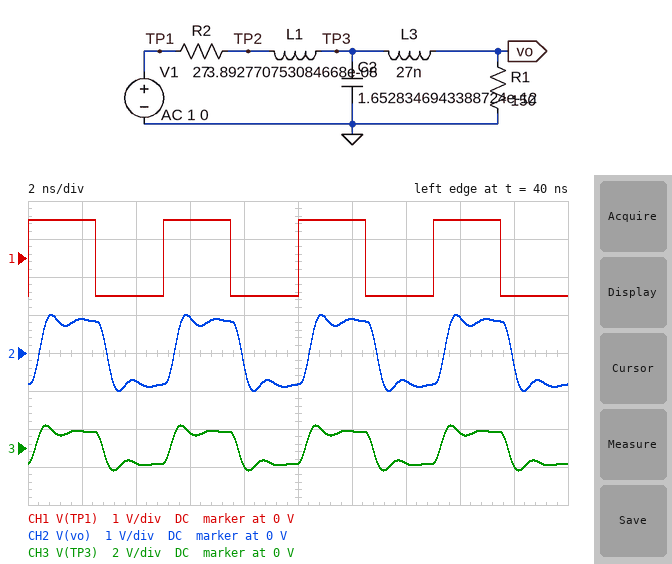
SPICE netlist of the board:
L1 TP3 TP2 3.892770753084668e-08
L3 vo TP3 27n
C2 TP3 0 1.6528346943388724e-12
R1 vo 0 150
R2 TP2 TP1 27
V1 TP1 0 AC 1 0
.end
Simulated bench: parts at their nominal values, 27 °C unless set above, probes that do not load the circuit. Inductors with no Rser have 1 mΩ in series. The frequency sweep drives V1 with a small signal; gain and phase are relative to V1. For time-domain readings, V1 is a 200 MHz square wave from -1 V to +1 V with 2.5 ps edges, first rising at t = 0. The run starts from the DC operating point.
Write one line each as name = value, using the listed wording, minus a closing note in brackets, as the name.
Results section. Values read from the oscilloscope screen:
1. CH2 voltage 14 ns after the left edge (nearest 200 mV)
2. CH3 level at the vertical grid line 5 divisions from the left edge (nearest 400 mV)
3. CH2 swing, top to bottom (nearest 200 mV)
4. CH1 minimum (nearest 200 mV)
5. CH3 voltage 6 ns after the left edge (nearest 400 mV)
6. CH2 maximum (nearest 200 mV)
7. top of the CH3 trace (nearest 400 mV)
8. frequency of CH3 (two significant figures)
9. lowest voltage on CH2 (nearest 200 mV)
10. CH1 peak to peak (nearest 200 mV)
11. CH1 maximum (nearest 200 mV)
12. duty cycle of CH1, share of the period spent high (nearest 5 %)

CH2 voltage 14 ns after the left edge = -800 mV
CH3 level at the vertical grid line 5 divisions from the left edge = -800 mV
CH2 swing, top to bottom = 2.0 V
CH1 minimum = -1.0 V
CH3 voltage 6 ns after the left edge = 800 mV
CH2 maximum = 1.0 V
top of the CH3 trace = 1.2 V
frequency of CH3 = 200 MHz
lowest voltage on CH2 = -1.0 V
CH1 peak to peak = 2.0 V
CH1 maximum = 1.0 V
duty cycle of CH1, share of the period spent high = 50 %
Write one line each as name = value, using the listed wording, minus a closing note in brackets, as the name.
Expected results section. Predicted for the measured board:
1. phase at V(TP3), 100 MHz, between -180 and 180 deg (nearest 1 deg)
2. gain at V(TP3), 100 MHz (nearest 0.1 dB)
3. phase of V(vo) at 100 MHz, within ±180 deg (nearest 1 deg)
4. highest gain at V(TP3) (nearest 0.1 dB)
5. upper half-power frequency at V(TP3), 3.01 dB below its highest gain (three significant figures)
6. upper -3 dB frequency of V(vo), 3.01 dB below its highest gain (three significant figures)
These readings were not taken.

phase at V(TP3), 100 MHz, between -180 and 180 deg = -8 deg
gain at V(TP3), 100 MHz = -1.5 dB
phase of V(vo) at 100 MHz, within ±180 deg = -15 deg
highest gain at V(TP3) = 1.3 dB
upper half-power frequency at V(TP3), 3.01 dB below its highest gain = 1.03 GHz
upper -3 dB frequency of V(vo), 3.01 dB below its highest gain = 988 MHz
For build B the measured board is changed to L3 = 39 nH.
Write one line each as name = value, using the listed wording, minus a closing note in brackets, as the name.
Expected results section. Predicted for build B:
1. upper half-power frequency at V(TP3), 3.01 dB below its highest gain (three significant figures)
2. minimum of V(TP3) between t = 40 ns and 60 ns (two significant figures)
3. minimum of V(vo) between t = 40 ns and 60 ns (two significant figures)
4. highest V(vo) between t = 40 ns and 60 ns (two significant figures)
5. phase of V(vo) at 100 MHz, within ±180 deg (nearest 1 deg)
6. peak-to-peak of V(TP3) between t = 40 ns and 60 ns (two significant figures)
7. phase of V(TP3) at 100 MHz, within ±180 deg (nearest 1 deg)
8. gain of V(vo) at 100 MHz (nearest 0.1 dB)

upper half-power frequency at V(TP3), 3.01 dB below its highest gain = 965 MHz
minimum of V(TP3) between t = 40 ns and 60 ns = -1.3 V
minimum of V(vo) between t = 40 ns and 60 ns = -960 mV
highest V(vo) between t = 40 ns and 60 ns = 960 mV
phase of V(vo) at 100 MHz, within ±180 deg = -17 deg
peak-to-peak of V(TP3) between t = 40 ns and 60 ns = 2.6 V
phase of V(TP3) at 100 MHz, within ±180 deg = -8 deg
gain of V(vo) at 100 MHz = -1.6 dB
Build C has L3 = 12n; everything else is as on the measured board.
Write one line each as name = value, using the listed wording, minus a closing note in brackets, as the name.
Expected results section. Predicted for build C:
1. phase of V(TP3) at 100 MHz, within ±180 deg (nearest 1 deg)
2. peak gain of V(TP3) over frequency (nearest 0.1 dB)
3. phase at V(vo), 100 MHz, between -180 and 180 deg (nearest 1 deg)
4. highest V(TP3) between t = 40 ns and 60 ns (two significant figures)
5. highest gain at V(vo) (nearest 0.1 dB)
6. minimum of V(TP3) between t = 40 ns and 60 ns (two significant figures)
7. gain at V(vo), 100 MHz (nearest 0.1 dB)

phase of V(TP3) at 100 MHz, within ±180 deg = -9 deg
peak gain of V(TP3) over frequency = -1.1 dB
phase at V(vo), 100 MHz, between -180 and 180 deg = -12 deg
highest V(TP3) between t = 40 ns and 60 ns = 1.0 V
highest gain at V(vo) = -1.3 dB
minimum of V(TP3) between t = 40 ns and 60 ns = -1.0 V
gain at V(vo), 100 MHz = -1.4 dB
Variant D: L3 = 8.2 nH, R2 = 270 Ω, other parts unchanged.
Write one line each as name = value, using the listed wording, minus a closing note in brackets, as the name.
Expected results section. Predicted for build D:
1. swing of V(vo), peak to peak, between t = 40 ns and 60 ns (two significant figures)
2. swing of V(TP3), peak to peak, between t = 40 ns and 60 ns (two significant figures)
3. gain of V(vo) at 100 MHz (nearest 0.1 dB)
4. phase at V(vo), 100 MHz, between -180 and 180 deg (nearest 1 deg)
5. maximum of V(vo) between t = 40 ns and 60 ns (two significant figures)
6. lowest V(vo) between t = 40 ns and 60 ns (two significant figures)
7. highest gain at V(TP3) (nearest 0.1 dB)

swing of V(vo), peak to peak, between t = 40 ns and 60 ns = 740 mV
swing of V(TP3), peak to peak, between t = 40 ns and 60 ns = 750 mV
gain of V(vo) at 100 MHz = -9.0 dB
phase at V(vo), 100 MHz, between -180 and 180 deg = -10 deg
maximum of V(vo) between t = 40 ns and 60 ns = 370 mV
lowest V(vo) between t = 40 ns and 60 ns = -370 mV
highest gain at V(TP3) = -8.9 dB
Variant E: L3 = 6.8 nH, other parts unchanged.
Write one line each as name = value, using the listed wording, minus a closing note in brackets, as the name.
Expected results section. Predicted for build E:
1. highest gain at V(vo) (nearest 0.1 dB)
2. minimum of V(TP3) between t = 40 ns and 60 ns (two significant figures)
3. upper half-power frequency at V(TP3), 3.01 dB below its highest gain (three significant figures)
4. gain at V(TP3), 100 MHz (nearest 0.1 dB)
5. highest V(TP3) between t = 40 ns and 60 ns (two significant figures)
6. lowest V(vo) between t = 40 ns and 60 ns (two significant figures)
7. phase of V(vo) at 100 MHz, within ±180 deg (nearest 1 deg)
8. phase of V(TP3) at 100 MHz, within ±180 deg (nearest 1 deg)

highest gain at V(vo) = -1.0 dB
minimum of V(TP3) between t = 40 ns and 60 ns = -1.0 V
upper half-power frequency at V(TP3), 3.01 dB below its highest gain = 865 MHz
gain at V(TP3), 100 MHz = -1.4 dB
highest V(TP3) between t = 40 ns and 60 ns = 1.0 V
lowest V(vo) between t = 40 ns and 60 ns = -1.0 V
phase of V(vo) at 100 MHz, within ±180 deg = -11 deg
phase of V(TP3) at 100 MHz, within ±180 deg = -9 deg
